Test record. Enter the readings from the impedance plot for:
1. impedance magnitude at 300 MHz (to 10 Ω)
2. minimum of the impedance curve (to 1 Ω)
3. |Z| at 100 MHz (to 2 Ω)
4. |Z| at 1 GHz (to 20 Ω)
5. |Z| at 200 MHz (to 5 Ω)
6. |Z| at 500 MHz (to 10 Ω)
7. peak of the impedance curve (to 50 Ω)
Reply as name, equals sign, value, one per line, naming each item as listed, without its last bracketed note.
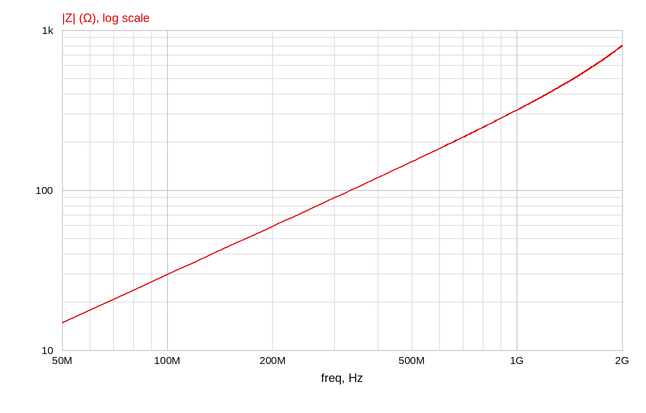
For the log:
impedance magnitude at 300 MHz = 90 Ω
minimum of the impedance curve = 15 Ω
|Z| at 100 MHz = 30 Ω
|Z| at 1 GHz = 320 Ω
|Z| at 200 MHz = 60 Ω
|Z| at 500 MHz = 150 Ω
peak of the impedance curve = 800 Ω
